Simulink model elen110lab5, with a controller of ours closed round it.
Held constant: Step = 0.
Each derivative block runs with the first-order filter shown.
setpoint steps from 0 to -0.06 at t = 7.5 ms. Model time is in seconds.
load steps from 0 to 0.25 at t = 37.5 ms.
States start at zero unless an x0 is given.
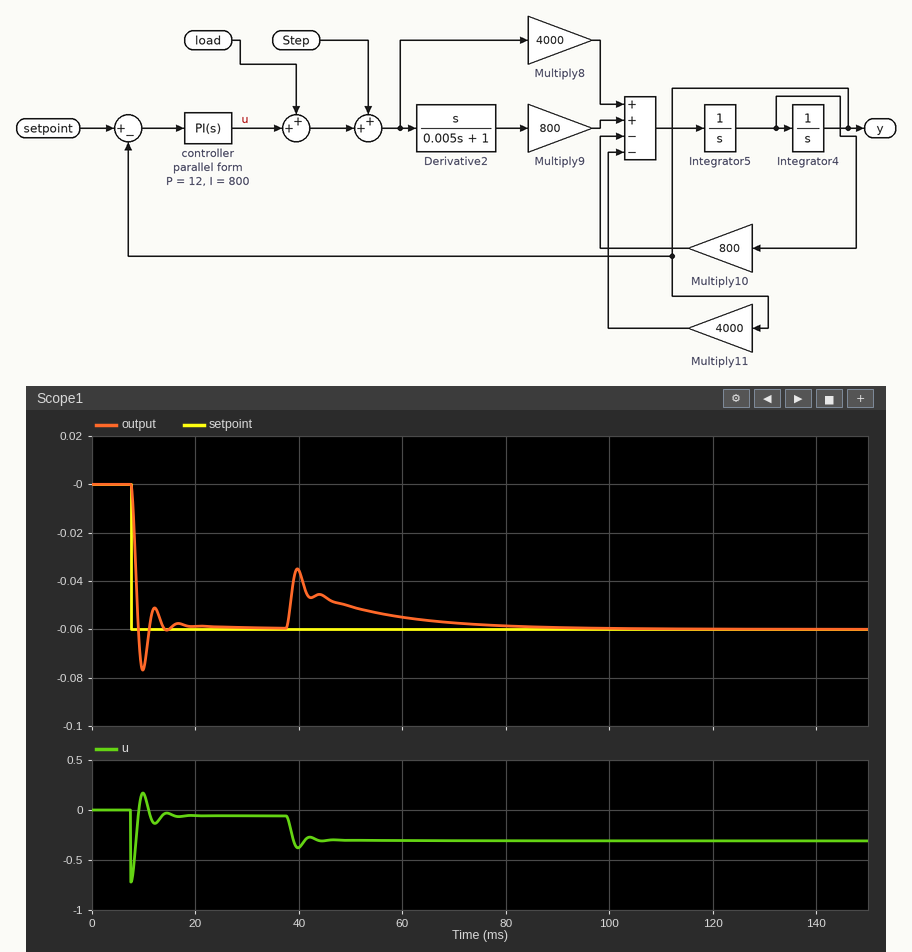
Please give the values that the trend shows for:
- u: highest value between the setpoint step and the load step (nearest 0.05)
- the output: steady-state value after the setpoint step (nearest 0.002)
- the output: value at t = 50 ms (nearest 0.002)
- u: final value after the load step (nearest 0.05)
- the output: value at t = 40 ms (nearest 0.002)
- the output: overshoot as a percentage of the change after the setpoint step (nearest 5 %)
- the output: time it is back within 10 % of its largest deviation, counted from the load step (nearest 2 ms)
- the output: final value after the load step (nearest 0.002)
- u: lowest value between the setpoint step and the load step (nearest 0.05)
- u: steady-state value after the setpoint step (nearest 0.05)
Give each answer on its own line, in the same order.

0.15
-0.060
-0.050
-0.30
-0.036
30 %
34 ms
-0.060
-0.70
-0.05
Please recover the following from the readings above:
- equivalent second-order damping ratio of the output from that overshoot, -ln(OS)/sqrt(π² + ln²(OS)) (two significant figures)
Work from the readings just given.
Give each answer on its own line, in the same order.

0.36
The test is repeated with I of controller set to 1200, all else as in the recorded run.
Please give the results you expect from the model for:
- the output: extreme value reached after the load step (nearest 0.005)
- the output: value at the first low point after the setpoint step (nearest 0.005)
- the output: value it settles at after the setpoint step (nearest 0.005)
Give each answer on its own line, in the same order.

-0.035
-0.080
-0.060
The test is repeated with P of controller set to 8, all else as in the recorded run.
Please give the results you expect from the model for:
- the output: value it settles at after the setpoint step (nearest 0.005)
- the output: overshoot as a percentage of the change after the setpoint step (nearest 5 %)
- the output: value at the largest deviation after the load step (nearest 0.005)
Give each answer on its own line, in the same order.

-0.060
20 %
-0.025
